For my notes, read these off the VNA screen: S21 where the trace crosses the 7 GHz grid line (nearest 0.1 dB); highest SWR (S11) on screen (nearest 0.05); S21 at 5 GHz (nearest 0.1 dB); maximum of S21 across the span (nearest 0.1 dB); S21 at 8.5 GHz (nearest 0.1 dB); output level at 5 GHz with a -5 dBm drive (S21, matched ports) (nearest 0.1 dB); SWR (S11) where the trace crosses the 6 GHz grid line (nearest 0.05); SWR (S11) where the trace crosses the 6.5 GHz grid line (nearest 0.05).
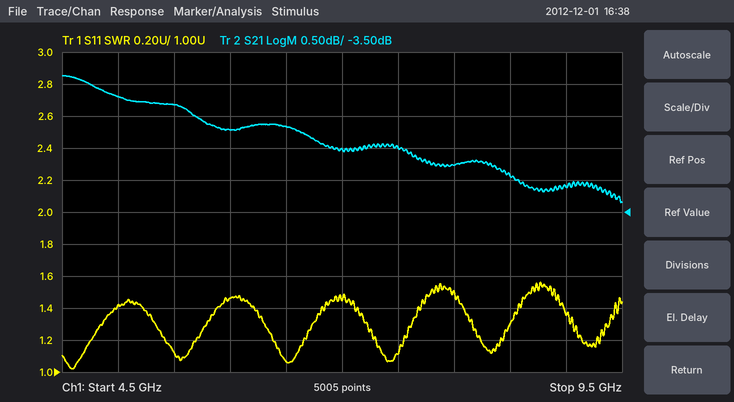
-2.5 dB
1.55
-1.7 dB
-1.4 dB
-2.9 dB
-6.7 dBm
1.45
1.05
